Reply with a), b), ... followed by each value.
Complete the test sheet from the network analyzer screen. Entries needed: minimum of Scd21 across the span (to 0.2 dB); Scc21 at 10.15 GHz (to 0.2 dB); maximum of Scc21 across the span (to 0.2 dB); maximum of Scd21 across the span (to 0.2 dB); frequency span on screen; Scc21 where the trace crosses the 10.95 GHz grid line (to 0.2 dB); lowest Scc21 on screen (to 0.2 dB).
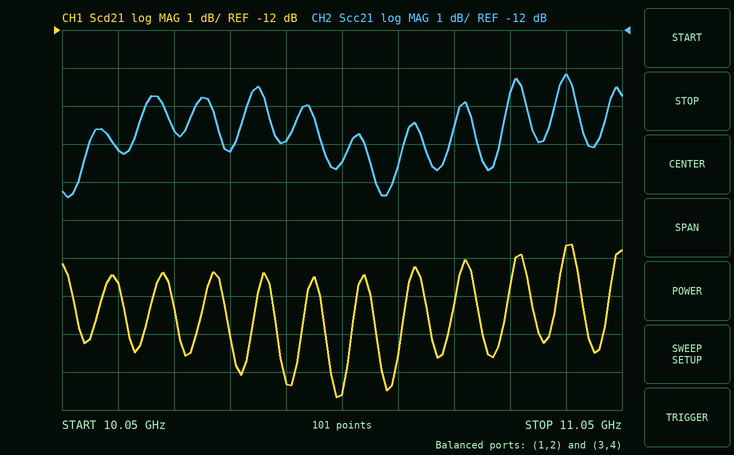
a) -21.6 dB
b) -15.2 dB
c) -13.2 dB
d) -17.6 dB
e) 1 GHz
f) -13.2 dB
g) -16.4 dB
